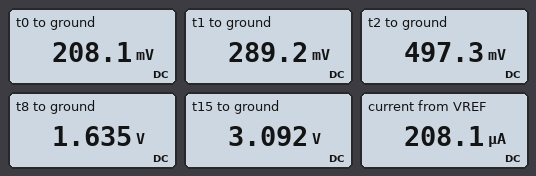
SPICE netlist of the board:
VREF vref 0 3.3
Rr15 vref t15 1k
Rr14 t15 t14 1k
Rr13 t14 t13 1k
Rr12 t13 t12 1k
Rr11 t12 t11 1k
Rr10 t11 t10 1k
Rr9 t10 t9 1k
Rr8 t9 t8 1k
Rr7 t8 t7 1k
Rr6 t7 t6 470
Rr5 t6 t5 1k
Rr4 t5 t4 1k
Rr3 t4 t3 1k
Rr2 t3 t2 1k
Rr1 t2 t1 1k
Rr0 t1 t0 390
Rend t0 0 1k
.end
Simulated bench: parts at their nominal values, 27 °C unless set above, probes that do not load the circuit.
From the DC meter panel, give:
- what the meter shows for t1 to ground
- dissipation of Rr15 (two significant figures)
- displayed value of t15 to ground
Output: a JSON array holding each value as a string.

["289.2 mV", "43 µW", "3.092 V"]
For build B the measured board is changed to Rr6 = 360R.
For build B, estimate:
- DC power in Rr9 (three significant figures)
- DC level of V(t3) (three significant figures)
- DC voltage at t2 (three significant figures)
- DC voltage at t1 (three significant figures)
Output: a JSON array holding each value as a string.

["43.9 µW", "710 mV", "501 mV", "291 mV"]
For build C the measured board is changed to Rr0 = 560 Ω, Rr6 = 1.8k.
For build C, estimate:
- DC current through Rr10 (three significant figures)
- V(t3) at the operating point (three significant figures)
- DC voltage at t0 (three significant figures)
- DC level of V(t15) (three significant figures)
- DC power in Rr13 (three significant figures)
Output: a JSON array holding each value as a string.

["190 µA", "677 mV", "190 mV", "3.11 V", "36.1 µW"]
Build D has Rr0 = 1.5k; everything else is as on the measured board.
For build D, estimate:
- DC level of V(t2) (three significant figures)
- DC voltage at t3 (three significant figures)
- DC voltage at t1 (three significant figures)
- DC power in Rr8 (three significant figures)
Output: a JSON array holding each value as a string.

["681 mV", "875 mV", "486 mV", "37.8 µW"]
